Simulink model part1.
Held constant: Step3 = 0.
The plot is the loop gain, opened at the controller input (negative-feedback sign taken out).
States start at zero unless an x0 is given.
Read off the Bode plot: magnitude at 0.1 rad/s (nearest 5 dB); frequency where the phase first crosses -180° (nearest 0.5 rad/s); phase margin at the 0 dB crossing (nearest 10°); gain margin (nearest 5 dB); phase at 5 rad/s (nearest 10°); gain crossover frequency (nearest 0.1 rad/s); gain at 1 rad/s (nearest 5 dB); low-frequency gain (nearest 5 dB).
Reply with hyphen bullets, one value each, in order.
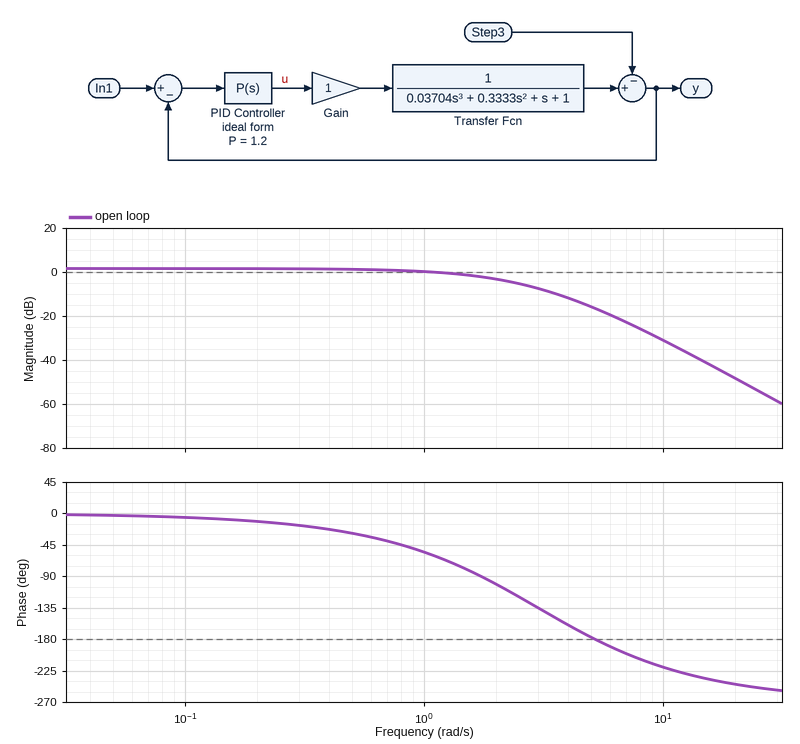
- 0 dB
- 5.0 rad/s
- 120°
- 15 dB
- -180°
- 1.1 rad/s
- 0 dB
- 0 dB
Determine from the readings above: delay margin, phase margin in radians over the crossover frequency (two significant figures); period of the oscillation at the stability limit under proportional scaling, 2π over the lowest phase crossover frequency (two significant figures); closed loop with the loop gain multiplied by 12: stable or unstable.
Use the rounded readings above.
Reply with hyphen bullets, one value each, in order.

- 1.9 s
- 1.3 s
- unstable
